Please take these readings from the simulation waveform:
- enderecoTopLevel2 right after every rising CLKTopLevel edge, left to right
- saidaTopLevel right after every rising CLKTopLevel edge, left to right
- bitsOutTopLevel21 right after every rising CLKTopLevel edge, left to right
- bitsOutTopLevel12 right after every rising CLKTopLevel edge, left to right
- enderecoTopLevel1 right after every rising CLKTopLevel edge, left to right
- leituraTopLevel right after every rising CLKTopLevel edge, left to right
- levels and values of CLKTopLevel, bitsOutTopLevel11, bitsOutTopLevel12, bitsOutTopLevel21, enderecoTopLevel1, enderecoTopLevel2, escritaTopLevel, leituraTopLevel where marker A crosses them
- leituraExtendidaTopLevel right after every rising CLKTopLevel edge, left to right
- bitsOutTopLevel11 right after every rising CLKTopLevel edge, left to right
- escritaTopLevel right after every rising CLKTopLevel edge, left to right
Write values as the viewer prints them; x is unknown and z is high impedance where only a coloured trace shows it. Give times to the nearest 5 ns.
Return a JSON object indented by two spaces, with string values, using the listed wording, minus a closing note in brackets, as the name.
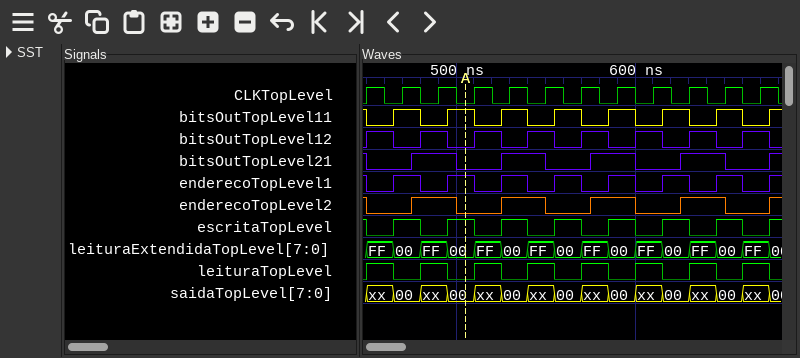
{
  "enderecoTopLevel2 right after every rising CLKTopLevel edge, left to right": "0 0 1 0 1 0 0 1 0 1 0 0",
  "saidaTopLevel right after every rising CLKTopLevel edge, left to right": "xx, 00, xx, xx, 00, xx, xx, 00, xx, xx, 00, xx",
  "bitsOutTopLevel21 right after every rising CLKTopLevel edge, left to right": "0 0 1 0 1 0 0 1 0 1 0 0",
  "bitsOutTopLevel12 right after every rising CLKTopLevel edge, left to right": "1 0 1 1 0 1 1 0 1 1 0 1",
  "enderecoTopLevel1 right after every rising CLKTopLevel edge, left to right": "0 1 0 0 1 0 0 1 0 0 1 0",
  "leituraTopLevel right after every rising CLKTopLevel edge, left to right": "1 0 1 1 0 1 1 0 1 1 0 1",
  "levels and values of CLKTopLevel, bitsOutTopLevel11, bitsOutTopLevel12, bitsOutTopLevel21, enderecoTopLevel1, enderecoTopLevel2, escritaTopLevel, leituraTopLevel where marker A crosses them": "CLKTopLevel=0, bitsOutTopLevel11=1, bitsOutTopLevel12=0, bitsOutTopLevel21=0, enderecoTopLevel1=1, enderecoTopLevel2=0, escritaTopLevel=1, leituraTopLevel=0",
  "leituraExtendidaTopLevel right after every rising CLKTopLevel edge, left to right": "FF, 00, FF, FF, 00, FF, FF, 00, FF, FF, 00, FF",
  "bitsOutTopLevel11 right after every rising CLKTopLevel edge, left to right": "0 1 0 0 1 0 0 1 0 0 1 0",
  "escritaTopLevel right after every rising CLKTopLevel edge, left to right": "0 1 0 0 1 0 0 1 0 0 1 0"
}
